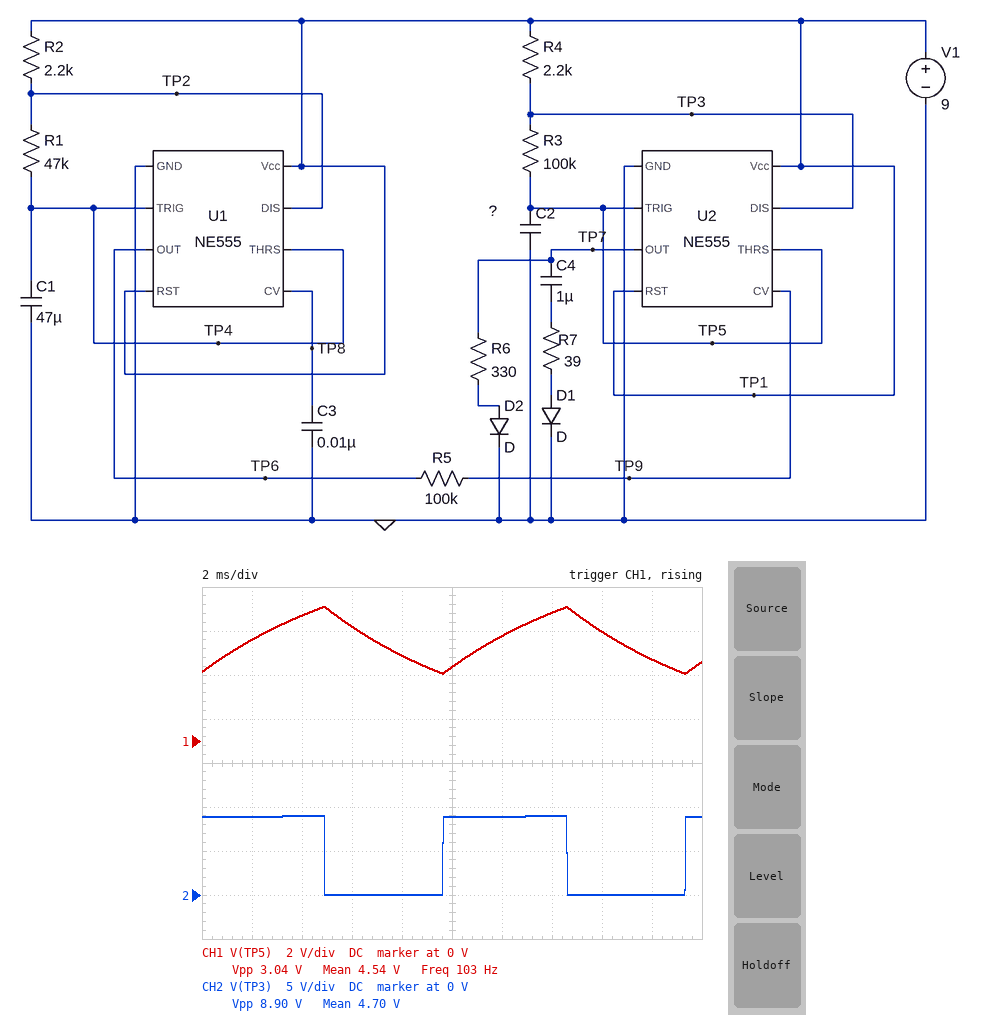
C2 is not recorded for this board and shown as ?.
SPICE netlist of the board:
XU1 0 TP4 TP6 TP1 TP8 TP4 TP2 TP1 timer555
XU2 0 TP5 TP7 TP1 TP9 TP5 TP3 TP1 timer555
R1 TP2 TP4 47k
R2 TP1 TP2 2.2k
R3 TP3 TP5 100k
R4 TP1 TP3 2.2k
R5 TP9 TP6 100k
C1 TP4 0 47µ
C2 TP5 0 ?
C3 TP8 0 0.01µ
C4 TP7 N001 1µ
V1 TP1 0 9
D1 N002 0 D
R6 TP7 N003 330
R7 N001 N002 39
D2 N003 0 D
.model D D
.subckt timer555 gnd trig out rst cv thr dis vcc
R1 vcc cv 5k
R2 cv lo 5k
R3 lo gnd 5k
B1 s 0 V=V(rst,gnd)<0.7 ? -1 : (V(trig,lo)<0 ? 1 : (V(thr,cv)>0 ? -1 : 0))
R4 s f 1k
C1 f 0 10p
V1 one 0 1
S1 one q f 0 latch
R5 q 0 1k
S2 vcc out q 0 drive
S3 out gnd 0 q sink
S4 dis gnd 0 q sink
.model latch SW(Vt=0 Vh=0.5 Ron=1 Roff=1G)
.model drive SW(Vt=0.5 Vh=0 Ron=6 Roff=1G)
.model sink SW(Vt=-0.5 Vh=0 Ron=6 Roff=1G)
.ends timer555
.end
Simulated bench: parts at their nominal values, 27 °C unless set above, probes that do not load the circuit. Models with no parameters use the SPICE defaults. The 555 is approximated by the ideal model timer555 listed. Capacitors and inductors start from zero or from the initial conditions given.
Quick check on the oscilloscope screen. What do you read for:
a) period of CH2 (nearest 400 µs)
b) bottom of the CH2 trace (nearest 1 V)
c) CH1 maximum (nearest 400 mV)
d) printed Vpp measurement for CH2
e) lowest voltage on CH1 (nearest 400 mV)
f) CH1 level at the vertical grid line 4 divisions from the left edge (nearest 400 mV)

9.6 ms
0 V
6.0 V
8.90 V
3.2 V
4.0 V
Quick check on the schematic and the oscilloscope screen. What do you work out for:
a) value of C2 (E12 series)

68 nF
